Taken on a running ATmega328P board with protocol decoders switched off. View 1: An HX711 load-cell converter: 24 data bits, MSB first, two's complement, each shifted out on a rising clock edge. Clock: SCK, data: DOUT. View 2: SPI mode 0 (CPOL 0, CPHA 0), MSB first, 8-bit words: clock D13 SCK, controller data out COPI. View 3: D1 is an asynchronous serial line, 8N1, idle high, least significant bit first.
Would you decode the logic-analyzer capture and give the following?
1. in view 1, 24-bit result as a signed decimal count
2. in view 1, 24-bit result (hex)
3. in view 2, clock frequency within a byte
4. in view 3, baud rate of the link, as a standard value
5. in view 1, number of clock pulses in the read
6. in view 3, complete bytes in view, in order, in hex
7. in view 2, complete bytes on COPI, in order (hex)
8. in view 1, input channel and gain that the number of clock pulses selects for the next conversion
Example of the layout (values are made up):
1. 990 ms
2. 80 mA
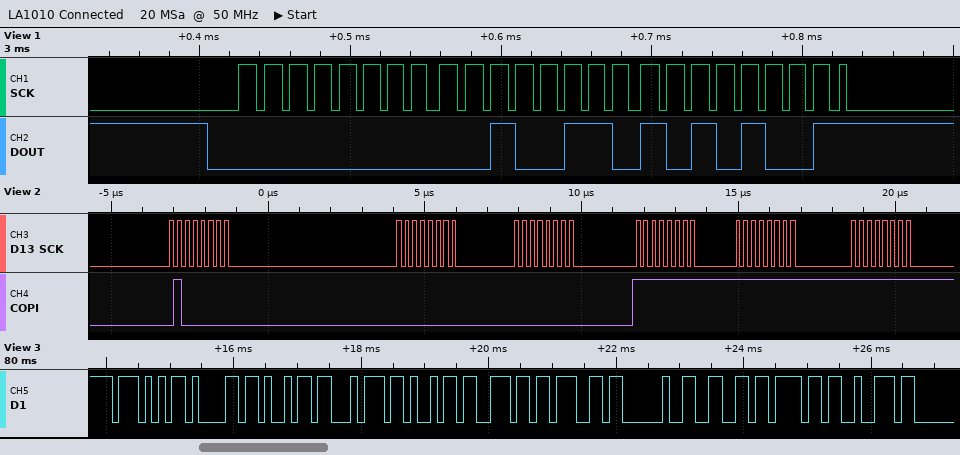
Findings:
1. 9897
2. 0x0026A9
3. 4 MHz
4. 9600 baud
5. 25
6. 0x57 0x61 0x69 0x74 0x69 0x6E 0x67 0x20 0x66 0x6F 0x72
7. 40 00 00 FF FF FF
8. channel A, gain 128
